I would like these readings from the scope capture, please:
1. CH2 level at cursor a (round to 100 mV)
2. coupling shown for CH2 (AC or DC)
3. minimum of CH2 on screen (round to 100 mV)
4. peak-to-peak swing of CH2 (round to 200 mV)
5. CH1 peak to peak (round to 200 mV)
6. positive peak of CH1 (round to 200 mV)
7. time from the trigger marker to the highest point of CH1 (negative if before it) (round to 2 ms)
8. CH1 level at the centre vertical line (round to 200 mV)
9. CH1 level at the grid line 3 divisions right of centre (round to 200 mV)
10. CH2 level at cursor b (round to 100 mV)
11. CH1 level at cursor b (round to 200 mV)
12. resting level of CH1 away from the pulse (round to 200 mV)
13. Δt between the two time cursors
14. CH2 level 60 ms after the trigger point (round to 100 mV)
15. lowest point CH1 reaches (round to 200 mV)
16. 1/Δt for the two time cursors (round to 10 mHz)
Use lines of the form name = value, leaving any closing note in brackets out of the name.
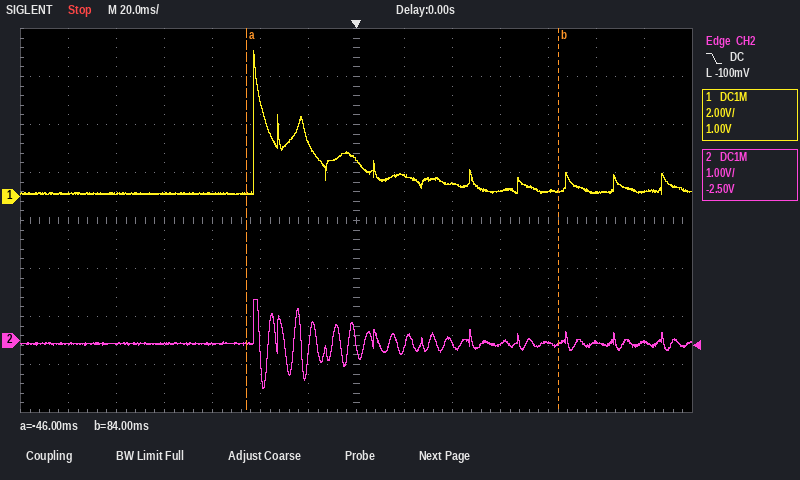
CH2 level at cursor a = -100 mV
coupling shown for CH2 = DC
minimum of CH2 on screen = -1.0 V
peak-to-peak swing of CH2 = 1.8 V
CH1 peak to peak = 6.0 V
positive peak of CH1 = 6.0 V
time from the trigger marker to the highest point of CH1 (negative if before it) = -42 ms
CH1 level at the centre vertical line = 1.6 V
CH1 level at the grid line 3 divisions right of centre = 200 mV
CH2 level at cursor b = -100 mV
CH1 level at cursor b = 200 mV
resting level of CH1 away from the pulse = 200 mV
Δt between the two time cursors = 130 ms
CH2 level 60 ms after the trigger point = -100 mV
lowest point CH1 reaches = 0.0 V
1/Δt for the two time cursors = 7.69 Hz
